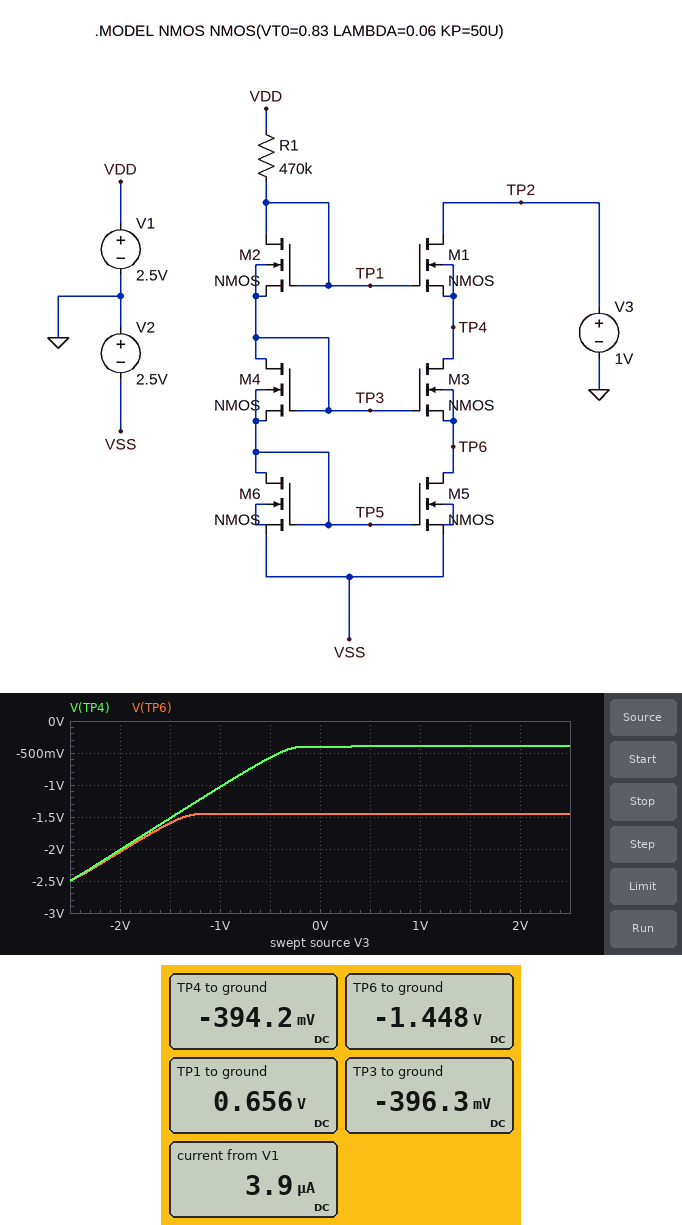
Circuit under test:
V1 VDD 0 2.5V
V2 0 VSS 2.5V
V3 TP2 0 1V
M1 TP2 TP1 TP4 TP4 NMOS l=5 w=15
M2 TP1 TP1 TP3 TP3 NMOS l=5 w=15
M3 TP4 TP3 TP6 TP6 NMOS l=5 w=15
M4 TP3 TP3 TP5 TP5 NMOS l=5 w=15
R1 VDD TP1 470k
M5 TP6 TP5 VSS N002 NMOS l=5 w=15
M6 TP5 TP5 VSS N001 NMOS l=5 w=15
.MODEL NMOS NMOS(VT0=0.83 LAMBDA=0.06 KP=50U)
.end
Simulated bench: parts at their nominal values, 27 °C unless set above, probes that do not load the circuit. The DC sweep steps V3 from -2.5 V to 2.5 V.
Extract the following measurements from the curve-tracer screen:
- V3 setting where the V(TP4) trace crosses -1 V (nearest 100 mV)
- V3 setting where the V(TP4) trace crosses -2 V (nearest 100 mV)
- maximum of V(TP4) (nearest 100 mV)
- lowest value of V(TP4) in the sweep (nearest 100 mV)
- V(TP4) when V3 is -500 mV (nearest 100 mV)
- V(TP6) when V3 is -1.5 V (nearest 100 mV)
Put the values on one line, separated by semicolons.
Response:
-1.0 V; -2.0 V; -400 mV; -2.5 V; -600 mV; -1.6 V
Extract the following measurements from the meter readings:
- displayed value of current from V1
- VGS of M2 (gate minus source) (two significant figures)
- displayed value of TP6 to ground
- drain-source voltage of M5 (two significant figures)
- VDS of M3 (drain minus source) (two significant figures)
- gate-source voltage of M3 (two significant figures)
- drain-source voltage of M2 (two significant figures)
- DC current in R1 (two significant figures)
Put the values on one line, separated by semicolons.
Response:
3.9 µA; 1.1 V; -1.448 V; 1.1 V; 1.1 V; 1.1 V; 1.1 V; 3.9 µA
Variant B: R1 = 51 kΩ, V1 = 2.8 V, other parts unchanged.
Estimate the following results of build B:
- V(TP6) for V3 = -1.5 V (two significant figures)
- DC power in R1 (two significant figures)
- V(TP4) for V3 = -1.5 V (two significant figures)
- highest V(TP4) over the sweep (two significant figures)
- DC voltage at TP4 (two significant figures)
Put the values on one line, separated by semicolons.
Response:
-1.7 V; 28 µW; -1.6 V; 250 mV; 230 mV
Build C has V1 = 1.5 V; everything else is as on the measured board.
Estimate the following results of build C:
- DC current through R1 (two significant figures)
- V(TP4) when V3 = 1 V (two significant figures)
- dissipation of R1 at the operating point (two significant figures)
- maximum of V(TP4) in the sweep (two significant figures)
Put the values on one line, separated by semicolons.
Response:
2.2 µA; -510 mV; 2.2 µW; -500 mV
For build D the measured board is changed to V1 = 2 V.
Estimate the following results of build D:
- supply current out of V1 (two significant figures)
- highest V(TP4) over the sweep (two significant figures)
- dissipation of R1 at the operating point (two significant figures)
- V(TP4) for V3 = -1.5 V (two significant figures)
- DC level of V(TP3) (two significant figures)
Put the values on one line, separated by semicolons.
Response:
3.0 µA; -440 mV; 4.3 µW; -1.5 V; -450 mV
